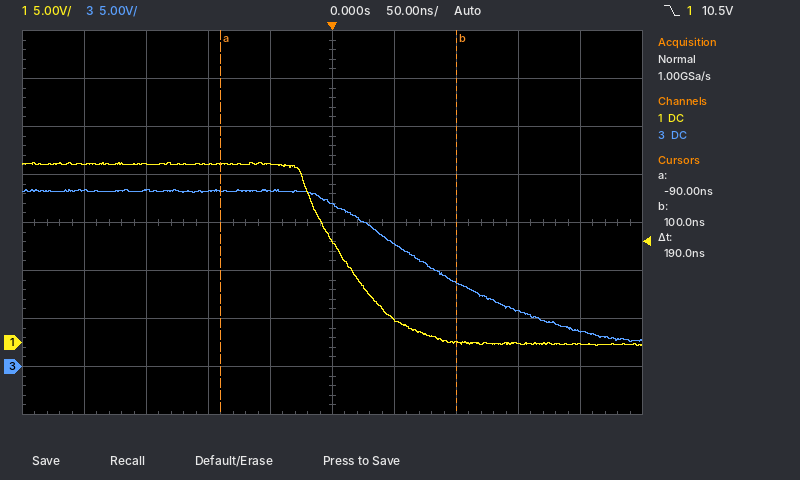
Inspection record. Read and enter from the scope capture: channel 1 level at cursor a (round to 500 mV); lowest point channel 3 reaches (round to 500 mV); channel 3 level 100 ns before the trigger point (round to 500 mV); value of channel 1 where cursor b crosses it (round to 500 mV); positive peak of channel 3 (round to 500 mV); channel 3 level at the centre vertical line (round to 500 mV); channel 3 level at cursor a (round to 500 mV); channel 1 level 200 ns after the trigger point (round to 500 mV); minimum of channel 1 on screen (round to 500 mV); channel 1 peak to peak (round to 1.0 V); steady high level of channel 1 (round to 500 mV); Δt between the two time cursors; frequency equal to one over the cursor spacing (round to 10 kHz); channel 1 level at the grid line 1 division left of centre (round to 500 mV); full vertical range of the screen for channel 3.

18.5 V
2.5 V
18.5 V
0.0 V
18.5 V
17.0 V
18.5 V
0.0 V
-500 mV
19.0 V
18.5 V
190 ns
5.26 MHz
18.5 V
40 V
